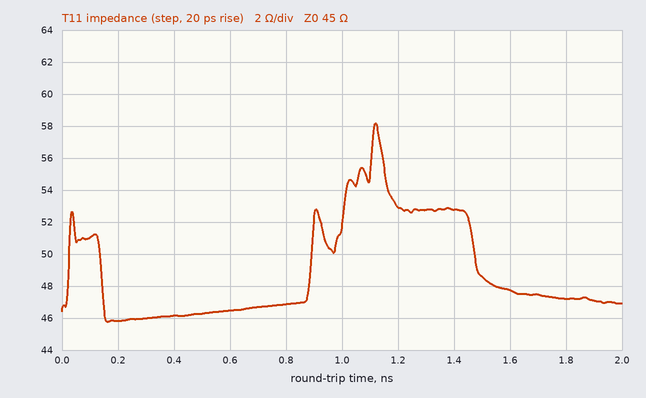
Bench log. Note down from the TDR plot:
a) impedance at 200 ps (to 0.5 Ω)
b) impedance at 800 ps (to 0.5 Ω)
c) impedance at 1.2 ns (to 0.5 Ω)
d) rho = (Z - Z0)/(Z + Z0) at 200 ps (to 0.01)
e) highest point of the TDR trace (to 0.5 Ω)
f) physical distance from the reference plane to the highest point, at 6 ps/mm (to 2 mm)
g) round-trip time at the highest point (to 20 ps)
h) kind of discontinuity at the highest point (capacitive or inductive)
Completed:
46.0 Ω
47.0 Ω
53.0 Ω
+0.01
58.0 Ω
94 mm
1.12 ns
inductive
